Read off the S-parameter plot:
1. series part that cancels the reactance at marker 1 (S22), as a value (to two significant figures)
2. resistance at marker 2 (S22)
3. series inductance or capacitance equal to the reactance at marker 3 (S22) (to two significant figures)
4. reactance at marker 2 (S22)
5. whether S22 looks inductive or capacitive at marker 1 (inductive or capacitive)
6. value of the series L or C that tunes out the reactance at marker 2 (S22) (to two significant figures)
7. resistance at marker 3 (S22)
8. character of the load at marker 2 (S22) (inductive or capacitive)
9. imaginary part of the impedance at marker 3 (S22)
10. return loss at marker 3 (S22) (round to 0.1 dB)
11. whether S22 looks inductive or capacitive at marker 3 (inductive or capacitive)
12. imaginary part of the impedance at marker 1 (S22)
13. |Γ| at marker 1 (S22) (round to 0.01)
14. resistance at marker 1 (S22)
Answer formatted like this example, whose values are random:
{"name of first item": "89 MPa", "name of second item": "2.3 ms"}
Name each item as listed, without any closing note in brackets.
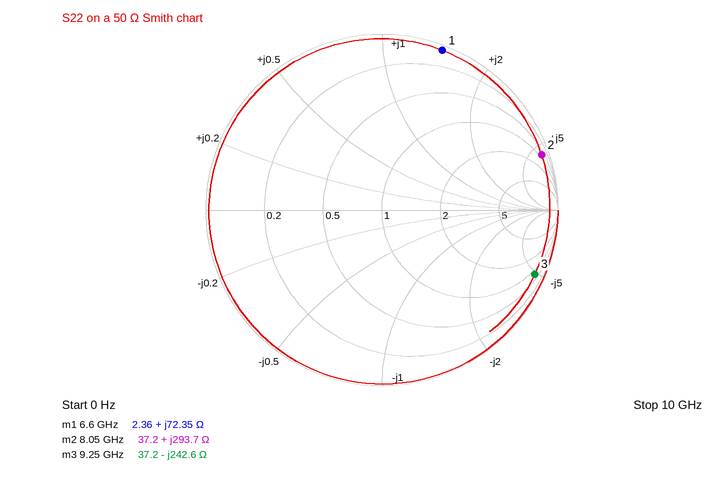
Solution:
{"series part that cancels the reactance at marker 1 (S22), as a value": "330 fF", "resistance at marker 2": "37.2 Ω", "series inductance or capacitance equal to the reactance at marker 3 (S22)": "71 fF", "reactance at marker 2": "+293.7 Ω", "whether S22 looks inductive or capacitive at marker 1": "inductive", "value of the series L or C that tunes out the reactance at marker 2 (S22)": "67 fF", "resistance at marker 3": "37.2 Ω", "character of the load at marker 2 (S22)": "inductive", "imaginary part of the impedance at marker 3": "-242.6 Ω", "return loss at marker 3 (S22)": "0.5 dB", "whether S22 looks inductive or capacitive at marker 3": "capacitive", "imaginary part of the impedance at marker 1": "+72.35 Ω", "|Γ| at marker 1 (S22)": "0.97", "resistance at marker 1": "2.36 Ω"}
